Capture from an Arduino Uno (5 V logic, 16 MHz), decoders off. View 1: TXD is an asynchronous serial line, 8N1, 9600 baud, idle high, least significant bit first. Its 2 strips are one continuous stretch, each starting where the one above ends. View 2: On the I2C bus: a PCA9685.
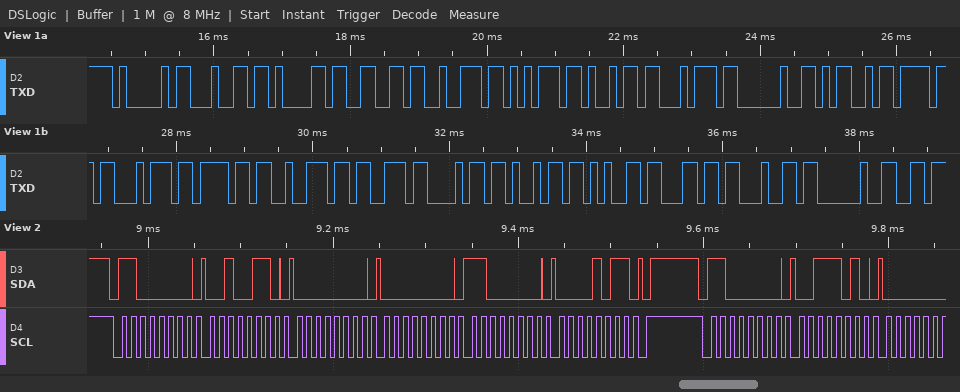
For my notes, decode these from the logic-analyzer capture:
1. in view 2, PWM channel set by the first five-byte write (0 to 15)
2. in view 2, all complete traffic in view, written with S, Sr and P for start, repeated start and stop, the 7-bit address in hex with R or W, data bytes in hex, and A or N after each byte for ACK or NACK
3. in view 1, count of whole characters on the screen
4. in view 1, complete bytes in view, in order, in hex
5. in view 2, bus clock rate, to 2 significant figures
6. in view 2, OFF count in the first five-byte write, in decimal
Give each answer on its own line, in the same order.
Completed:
8
S 60W A 26 A 00 A 00 A C0 A 0B A P S 60W A 3A A
21
41 64 61 66 72 75 69 74 20 4D 6F 74 6F 72 73 68 69 65 6C 64 20
100 kHz
3008
